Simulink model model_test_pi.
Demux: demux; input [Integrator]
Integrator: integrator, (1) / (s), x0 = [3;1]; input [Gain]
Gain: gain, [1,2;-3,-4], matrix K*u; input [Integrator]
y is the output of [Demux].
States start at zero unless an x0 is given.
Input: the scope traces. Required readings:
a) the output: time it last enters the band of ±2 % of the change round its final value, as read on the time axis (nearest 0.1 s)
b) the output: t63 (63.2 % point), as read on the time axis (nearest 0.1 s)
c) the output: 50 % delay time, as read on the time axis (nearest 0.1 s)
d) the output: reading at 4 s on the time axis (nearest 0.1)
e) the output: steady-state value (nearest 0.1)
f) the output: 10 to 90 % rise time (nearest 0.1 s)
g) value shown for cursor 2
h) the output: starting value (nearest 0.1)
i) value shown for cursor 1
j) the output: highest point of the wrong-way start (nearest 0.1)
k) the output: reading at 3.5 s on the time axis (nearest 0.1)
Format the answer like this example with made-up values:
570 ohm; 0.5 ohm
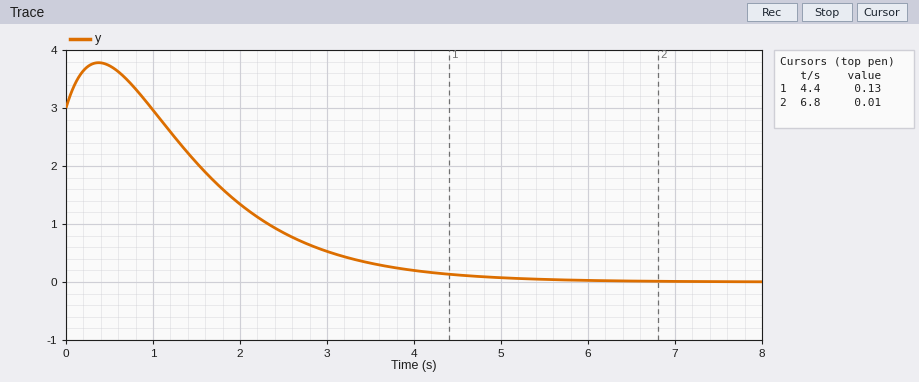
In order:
5.2 s; 2.2 s; 1.9 s; 0.2; 0.0; 2.4 s; 0.01; 3.0; 0.13; 3.8; 0.3
